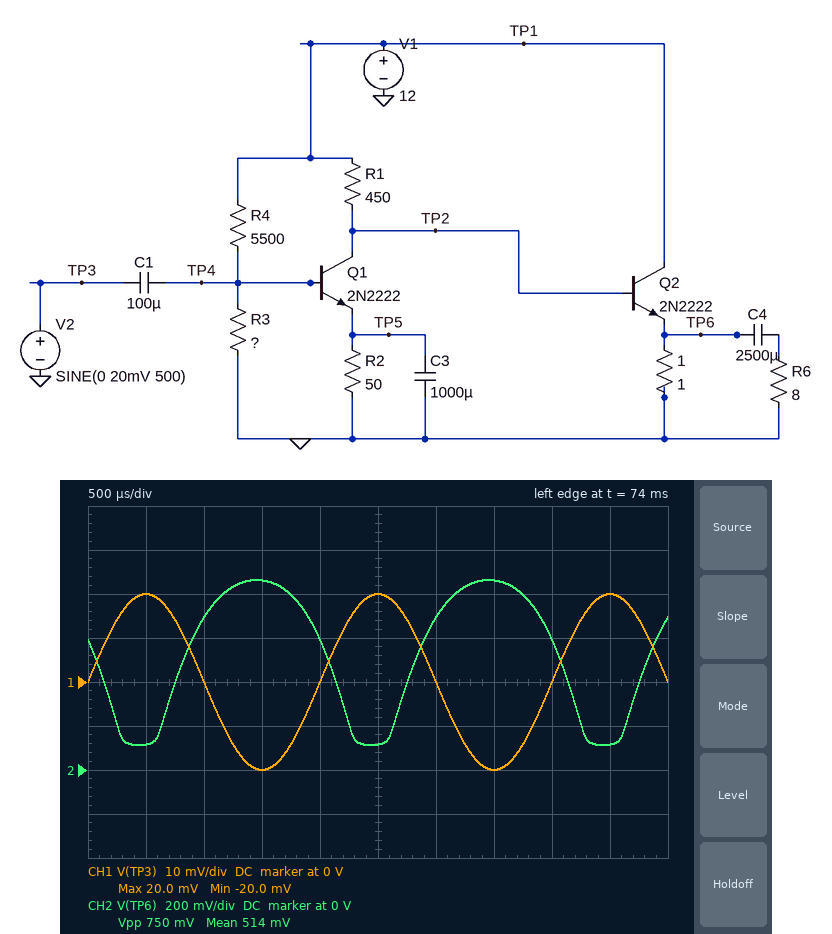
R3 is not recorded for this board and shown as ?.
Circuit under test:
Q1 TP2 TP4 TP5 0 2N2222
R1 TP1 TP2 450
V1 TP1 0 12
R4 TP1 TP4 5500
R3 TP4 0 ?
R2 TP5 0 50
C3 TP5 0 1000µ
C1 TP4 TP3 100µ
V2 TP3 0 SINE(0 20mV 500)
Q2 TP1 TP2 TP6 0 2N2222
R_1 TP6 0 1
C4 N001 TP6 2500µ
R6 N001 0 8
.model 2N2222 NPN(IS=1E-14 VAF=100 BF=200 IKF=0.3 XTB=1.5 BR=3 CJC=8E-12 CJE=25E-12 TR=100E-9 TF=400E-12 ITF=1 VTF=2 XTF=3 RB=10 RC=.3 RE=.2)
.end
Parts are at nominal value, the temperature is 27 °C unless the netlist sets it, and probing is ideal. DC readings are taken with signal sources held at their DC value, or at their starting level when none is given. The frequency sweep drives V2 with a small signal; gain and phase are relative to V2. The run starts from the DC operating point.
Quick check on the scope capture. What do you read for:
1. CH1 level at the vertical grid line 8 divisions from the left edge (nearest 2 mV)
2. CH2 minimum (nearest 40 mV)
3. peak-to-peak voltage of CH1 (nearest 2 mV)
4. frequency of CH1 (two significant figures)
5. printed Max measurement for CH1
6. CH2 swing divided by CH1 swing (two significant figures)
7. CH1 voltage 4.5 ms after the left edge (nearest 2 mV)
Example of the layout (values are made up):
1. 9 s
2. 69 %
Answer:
1. 0 V
2. 120 mV
3. 40 mV
4. 500 Hz
5. 20.0 mV
6. 19
7. 20 mV
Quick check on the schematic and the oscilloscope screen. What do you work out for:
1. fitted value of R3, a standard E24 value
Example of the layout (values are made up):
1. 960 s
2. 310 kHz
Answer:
1. 820 Ω
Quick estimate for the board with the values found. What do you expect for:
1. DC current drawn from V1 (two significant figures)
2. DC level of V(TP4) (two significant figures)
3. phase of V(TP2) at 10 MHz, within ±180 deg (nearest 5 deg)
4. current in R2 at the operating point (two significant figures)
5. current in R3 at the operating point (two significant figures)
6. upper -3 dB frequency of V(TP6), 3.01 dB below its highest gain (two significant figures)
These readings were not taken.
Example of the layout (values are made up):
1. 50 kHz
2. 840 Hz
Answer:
1. 630 mA
2. 1.5 V
3. 130 deg
4. 15 mA
5. 1.8 mA
6. 7.5 MHz
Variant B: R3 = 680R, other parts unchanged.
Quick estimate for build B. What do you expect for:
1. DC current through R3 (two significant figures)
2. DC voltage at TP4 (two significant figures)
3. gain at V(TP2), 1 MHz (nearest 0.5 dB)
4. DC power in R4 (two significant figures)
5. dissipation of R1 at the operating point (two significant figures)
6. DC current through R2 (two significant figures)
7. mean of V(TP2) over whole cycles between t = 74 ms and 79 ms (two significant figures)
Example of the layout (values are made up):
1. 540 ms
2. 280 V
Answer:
1. 1.9 mA
2. 1.3 V
3. 25.5 dB
4. 21 mW
5. 230 mW
6. 11 mA
7. 1.9 V
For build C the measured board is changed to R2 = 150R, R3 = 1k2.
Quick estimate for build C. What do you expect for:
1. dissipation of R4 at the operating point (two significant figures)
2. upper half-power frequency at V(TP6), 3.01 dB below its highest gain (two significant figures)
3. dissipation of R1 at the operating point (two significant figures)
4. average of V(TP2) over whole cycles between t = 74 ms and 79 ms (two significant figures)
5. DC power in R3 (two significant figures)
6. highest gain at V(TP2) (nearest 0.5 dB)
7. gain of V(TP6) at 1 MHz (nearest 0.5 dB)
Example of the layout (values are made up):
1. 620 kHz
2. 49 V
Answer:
1. 18 mW
2. 9.5 MHz
3. 220 mW
4. 2.0 V
5. 3.7 mW
6. 23.5 dB
7. 19.5 dB
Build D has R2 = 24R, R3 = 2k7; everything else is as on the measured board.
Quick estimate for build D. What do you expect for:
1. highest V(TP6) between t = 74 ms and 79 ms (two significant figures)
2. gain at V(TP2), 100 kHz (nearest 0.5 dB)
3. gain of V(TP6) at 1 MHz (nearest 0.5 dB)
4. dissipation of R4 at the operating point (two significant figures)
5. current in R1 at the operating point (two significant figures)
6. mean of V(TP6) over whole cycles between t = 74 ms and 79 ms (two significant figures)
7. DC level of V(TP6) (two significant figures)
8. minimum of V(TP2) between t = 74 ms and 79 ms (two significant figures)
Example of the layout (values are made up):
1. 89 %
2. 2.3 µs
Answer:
1. 130 mV
2. 1.5 dB
3. -19.5 dB
4. 20 mW
5. 25 mA
6. 20 mV
7. 5.7 mV
8. 690 mV
